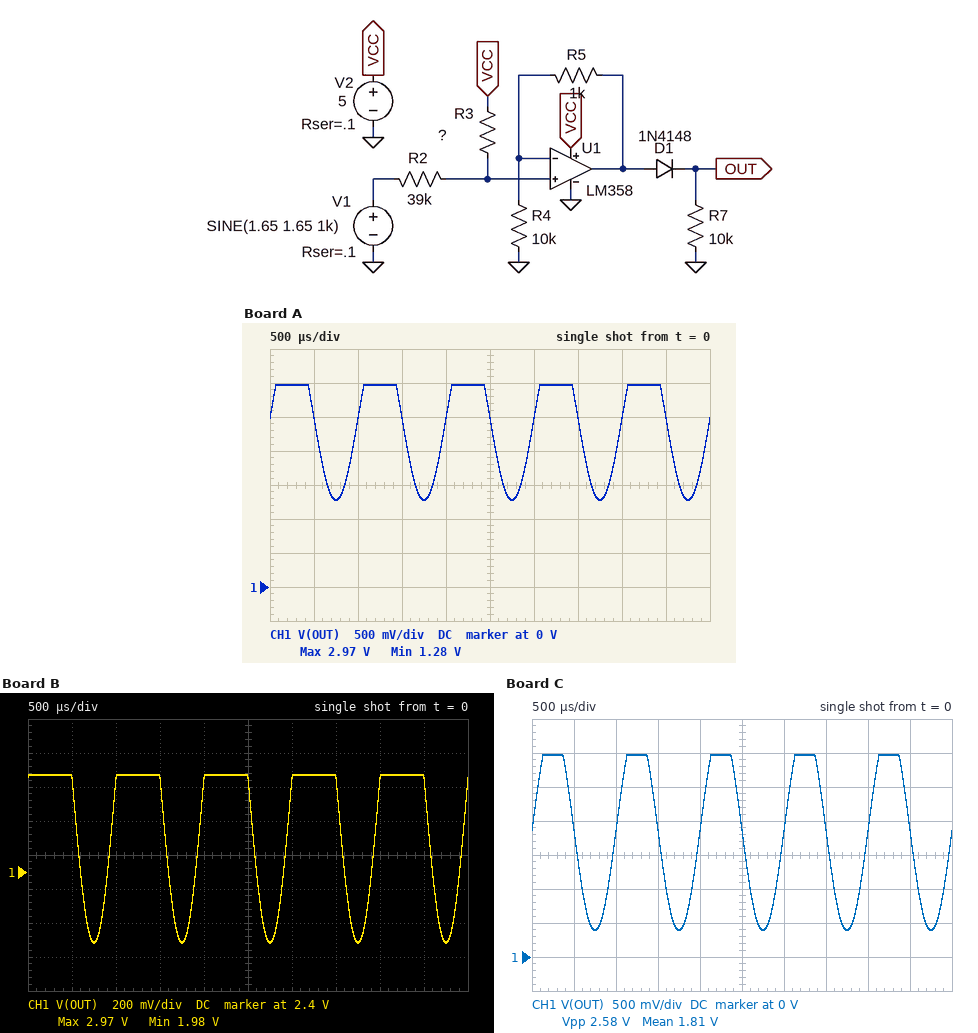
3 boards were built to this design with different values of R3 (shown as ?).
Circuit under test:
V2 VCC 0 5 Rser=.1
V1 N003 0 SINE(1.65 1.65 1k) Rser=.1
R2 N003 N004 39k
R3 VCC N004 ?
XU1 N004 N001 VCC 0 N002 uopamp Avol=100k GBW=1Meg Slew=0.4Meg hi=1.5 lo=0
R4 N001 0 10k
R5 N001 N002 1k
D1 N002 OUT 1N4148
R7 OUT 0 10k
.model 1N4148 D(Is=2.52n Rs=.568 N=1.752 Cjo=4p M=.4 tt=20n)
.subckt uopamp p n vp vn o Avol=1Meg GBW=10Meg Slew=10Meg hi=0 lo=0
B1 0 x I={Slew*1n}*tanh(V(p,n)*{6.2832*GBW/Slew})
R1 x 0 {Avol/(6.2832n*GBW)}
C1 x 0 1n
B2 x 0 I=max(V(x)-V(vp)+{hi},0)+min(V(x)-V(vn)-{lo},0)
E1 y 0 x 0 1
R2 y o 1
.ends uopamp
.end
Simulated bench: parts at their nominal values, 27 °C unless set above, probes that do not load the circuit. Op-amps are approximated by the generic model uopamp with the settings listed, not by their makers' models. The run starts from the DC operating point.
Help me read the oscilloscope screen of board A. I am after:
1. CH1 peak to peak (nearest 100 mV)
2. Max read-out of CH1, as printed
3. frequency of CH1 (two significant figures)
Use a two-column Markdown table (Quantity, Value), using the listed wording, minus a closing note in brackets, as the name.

| Quantity | Value |
|---|---|
| CH1 peak to peak | 1.7 V |
| Max read-out of CH1, as printed | 2.97 V |
| frequency of CH1 | 1.0 kHz |
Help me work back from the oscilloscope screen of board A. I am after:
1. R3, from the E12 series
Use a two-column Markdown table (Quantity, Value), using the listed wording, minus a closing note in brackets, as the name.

| Quantity | Value |
|---|---|
| R3, from the E12 series | 82 kΩ |
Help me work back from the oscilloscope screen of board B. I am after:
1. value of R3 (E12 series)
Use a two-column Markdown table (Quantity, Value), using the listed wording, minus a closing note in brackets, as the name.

| Quantity | Value |
|---|---|
| value of R3 | 47 kΩ |
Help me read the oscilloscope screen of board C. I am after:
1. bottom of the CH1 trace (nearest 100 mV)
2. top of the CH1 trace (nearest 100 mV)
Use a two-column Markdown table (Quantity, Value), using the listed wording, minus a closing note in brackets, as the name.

| Quantity | Value |
|---|---|
| bottom of the CH1 trace | 400 mV |
| top of the CH1 trace | 3.0 V |
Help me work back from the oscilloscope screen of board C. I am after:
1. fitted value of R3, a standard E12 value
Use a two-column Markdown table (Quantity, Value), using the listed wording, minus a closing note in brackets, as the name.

| Quantity | Value |
|---|---|
| fitted value of R3, a standard E12 value | 220 kΩ |
